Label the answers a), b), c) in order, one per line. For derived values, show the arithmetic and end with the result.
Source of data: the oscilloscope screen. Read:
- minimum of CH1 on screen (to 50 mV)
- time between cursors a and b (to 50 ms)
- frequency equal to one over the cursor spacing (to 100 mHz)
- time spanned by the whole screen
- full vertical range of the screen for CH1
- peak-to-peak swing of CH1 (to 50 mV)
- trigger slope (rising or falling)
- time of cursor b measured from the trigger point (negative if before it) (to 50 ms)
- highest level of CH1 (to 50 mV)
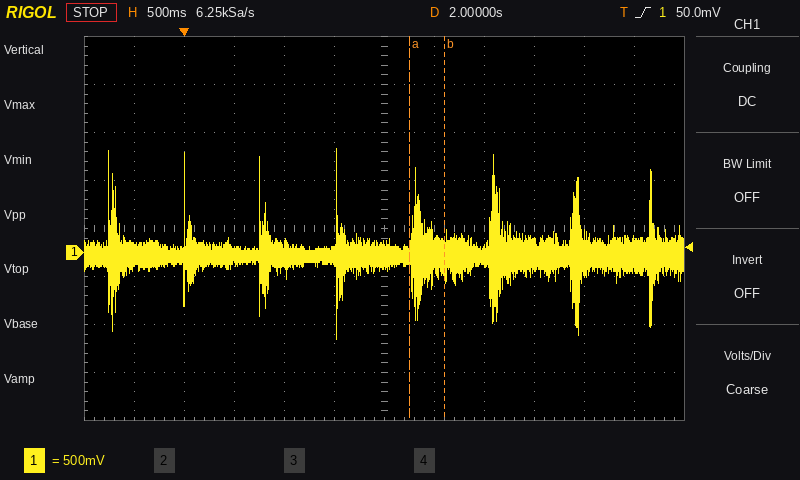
a) -900 mV
b) 350 ms
c) 1 / 350 ms ≈ 2.9 Hz
d) 6 s
e) 4 V
f) 1.10 V − (-900 mV) = 2.00 V
g) rising
h) +2.60 s
i) 1.10 V
